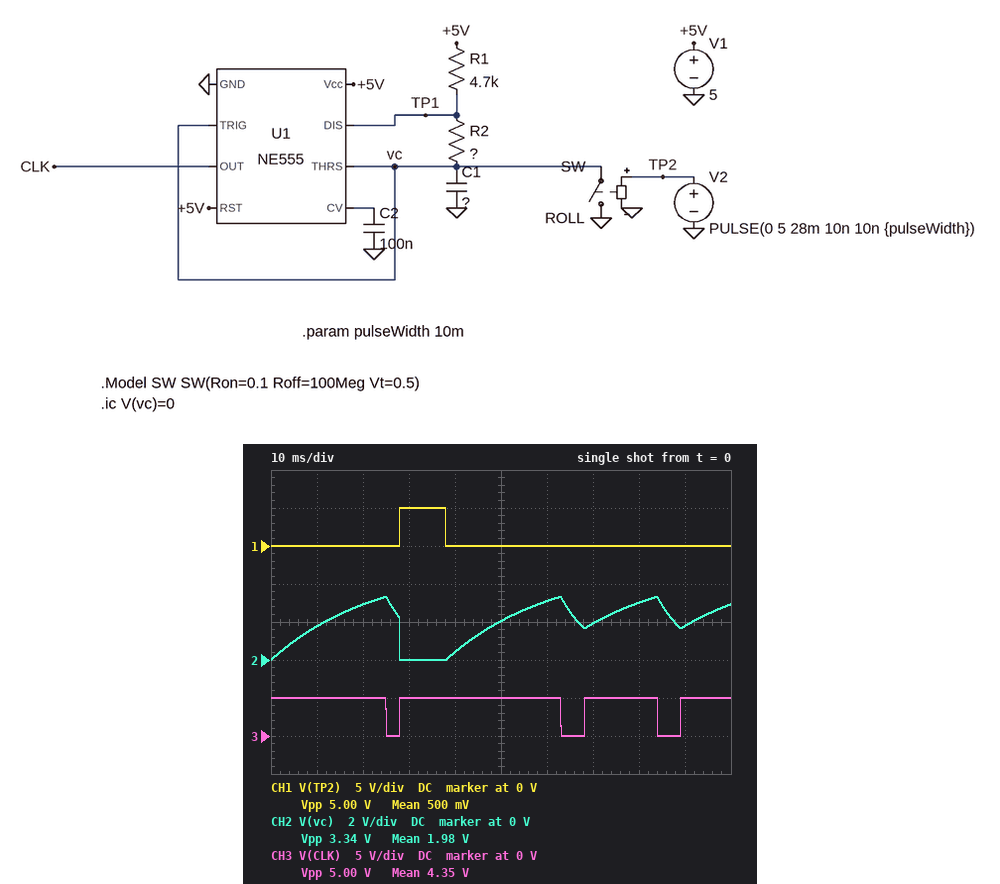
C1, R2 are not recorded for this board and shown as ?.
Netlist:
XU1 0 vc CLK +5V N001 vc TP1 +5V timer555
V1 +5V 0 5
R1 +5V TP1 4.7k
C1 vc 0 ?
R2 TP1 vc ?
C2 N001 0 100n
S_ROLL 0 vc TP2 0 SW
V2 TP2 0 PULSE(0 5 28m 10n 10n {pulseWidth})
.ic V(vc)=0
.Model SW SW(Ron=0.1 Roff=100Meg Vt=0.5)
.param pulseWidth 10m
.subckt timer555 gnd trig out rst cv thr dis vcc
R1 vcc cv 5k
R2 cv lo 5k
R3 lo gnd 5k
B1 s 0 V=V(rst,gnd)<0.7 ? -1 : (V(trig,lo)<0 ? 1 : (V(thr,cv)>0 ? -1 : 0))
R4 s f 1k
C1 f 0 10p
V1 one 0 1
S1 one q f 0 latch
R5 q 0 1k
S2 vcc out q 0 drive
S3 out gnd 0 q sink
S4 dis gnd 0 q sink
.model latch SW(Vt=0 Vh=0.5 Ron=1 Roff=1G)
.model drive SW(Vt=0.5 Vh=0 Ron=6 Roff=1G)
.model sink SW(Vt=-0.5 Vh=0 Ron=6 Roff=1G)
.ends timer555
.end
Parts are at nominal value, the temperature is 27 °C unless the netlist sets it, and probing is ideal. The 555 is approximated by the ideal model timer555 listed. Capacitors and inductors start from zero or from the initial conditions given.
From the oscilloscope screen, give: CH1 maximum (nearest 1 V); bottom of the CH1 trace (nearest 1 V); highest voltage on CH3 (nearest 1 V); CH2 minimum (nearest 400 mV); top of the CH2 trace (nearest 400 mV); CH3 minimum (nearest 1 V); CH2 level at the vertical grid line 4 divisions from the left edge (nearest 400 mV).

5 V
0 V
5 V
0 V
3.2 V
0 V
400 mV
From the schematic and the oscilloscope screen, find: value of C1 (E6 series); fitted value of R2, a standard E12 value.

3.3 µF
2.2 kΩ
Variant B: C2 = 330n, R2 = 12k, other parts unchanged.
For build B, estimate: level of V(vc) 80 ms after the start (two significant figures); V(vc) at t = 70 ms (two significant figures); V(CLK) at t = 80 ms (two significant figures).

2.7 V
2.2 V
5.0 V
